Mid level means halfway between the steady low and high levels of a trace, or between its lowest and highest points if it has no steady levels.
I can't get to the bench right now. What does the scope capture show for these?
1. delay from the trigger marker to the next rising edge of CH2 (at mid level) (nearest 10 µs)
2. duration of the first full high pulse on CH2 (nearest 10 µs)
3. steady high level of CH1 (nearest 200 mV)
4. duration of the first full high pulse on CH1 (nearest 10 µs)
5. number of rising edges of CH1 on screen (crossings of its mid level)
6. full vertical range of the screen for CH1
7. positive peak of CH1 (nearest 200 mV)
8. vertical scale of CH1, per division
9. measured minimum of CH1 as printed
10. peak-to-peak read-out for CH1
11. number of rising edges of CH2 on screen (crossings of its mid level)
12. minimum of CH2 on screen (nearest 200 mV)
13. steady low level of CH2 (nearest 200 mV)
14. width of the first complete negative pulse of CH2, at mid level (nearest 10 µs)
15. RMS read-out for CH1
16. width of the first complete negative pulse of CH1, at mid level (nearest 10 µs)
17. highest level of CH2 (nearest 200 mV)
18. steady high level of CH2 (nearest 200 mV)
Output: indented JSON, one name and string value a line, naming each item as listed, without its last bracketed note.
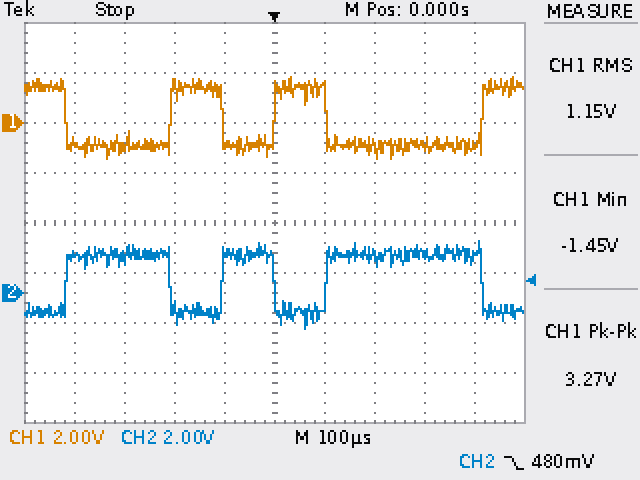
{
  "delay from the trigger marker to the next rising edge of CH2 (at mid level)": "100 µs",
  "duration of the first full high pulse on CH2": "210 µs",
  "steady high level of CH1": "1.4 V",
  "duration of the first full high pulse on CH1": "100 µs",
  "number of rising edges of CH1 on screen": "3",
  "full vertical range of the screen for CH1": "16 V",
  "positive peak of CH1": "1.8 V",
  "vertical scale of CH1, per division": "2 V",
  "measured minimum of CH1 as printed": "-1.45 V",
  "peak-to-peak read-out for CH1": "3.27 V",
  "number of rising edges of CH2 on screen": "3",
  "minimum of CH2 on screen": "-1.4 V",
  "steady low level of CH2": "-800 mV",
  "width of the first complete negative pulse of CH2, at mid level": "100 µs",
  "RMS read-out for CH1": "1.15 V",
  "width of the first complete negative pulse of CH1, at mid level": "210 µs",
  "highest level of CH2": "2.0 V",
  "steady high level of CH2": "1.6 V"
}
